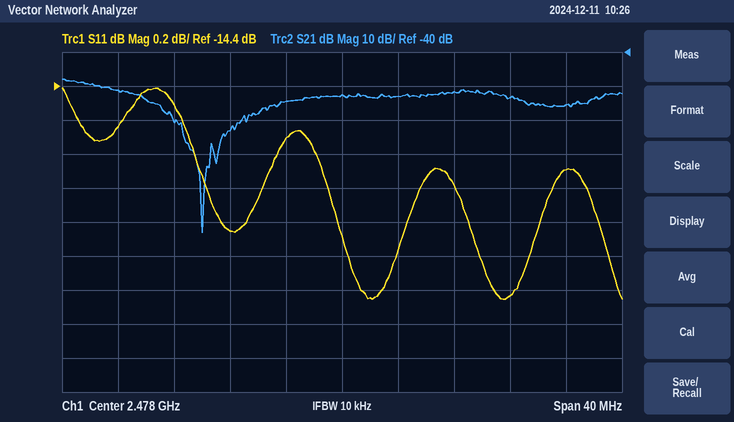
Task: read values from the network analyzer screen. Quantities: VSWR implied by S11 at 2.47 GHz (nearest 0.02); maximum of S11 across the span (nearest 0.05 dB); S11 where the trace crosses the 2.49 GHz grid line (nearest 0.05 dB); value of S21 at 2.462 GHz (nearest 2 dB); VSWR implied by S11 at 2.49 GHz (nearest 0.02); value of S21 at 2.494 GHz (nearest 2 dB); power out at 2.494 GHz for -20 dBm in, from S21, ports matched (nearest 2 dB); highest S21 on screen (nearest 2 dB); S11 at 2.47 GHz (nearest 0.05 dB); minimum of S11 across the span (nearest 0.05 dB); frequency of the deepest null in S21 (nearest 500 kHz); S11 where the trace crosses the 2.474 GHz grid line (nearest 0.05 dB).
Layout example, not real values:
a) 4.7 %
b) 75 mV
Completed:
a) 1.42
b) -14.40 dB
c) -15.65 dB
d) -52 dB
e) 1.40
f) -56 dB
g) -76 dBm
h) -48 dB
i) -15.25 dB
j) -15.65 dB
k) 2.4680 GHz
l) -14.70 dB
